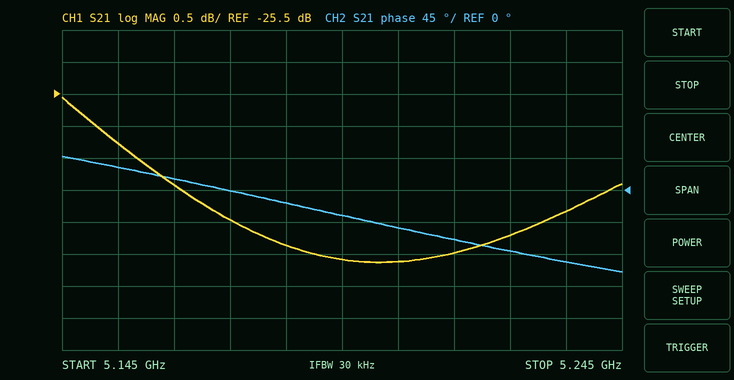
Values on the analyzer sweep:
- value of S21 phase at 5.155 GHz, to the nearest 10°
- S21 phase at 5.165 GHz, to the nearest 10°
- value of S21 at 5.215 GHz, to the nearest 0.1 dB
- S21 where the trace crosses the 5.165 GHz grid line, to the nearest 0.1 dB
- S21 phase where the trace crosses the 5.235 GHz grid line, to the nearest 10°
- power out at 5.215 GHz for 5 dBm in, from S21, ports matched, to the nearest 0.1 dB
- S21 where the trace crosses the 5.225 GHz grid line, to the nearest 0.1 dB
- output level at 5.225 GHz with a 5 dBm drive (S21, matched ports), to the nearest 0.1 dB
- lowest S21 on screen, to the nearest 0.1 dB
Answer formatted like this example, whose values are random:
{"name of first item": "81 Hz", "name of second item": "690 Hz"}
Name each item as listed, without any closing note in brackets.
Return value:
{"value of S21 phase at 5.155 GHz, to the nearest 10°": "30°", "S21 phase at 5.165 GHz, to the nearest 10°": "20°", "value of S21 at 5.215 GHz, to the nearest 0.1 dB": "-28.0 dB", "S21 where the trace crosses the 5.165 GHz grid line, to the nearest 0.1 dB": "-26.9 dB", "S21 phase where the trace crosses the 5.235 GHz grid line, to the nearest 10°": "-100°", "power out at 5.215 GHz for 5 dBm in, from S21, ports matched, to the nearest 0.1 dB": "-23.0 dBm", "S21 where the trace crosses the 5.225 GHz grid line, to the nearest 0.1 dB": "-27.7 dB", "output level at 5.225 GHz with a 5 dBm drive (S21, matched ports), to the nearest 0.1 dB": "-22.7 dBm", "lowest S21 on screen, to the nearest 0.1 dB": "-28.1 dB"}
